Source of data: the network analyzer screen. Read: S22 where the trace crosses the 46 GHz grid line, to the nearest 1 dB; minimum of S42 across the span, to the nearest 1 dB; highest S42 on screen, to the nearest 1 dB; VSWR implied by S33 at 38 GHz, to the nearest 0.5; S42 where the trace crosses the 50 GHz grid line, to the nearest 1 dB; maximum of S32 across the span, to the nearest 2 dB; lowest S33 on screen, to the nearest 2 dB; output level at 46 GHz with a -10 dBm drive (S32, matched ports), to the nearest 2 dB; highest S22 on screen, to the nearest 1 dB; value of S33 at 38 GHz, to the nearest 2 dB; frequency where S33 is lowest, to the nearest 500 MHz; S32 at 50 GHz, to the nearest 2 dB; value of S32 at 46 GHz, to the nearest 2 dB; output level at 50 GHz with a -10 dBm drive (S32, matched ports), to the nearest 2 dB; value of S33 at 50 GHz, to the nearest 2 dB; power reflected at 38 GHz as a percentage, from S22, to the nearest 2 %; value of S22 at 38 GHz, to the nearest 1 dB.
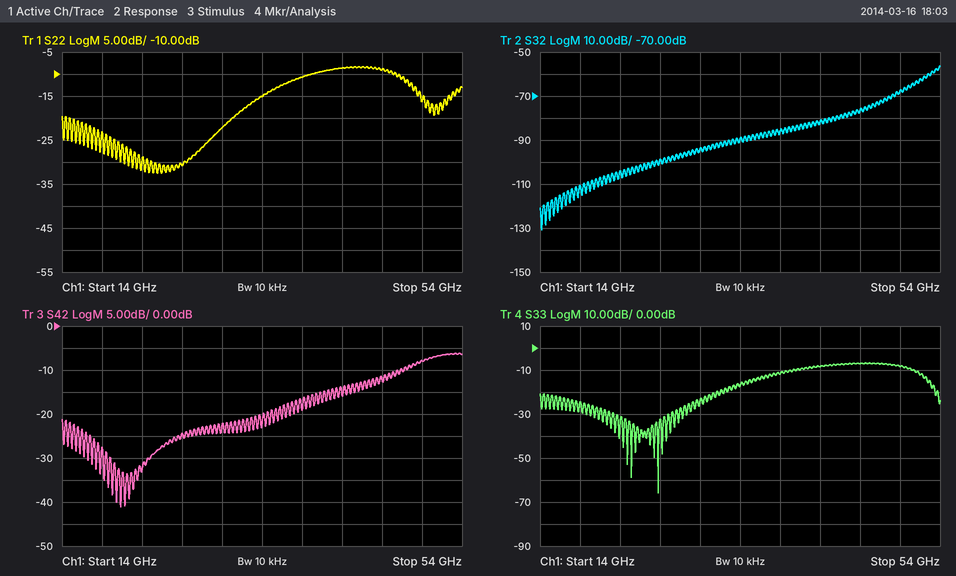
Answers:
-9 dB
-41 dB
-6 dB
1.5
-8 dB
-56 dB
-66 dB
-86 dBm
-8 dB
-12 dB
26.0 GHz
-68 dB
-76 dB
-78 dBm
-8 dB
8 %
-11 dB
